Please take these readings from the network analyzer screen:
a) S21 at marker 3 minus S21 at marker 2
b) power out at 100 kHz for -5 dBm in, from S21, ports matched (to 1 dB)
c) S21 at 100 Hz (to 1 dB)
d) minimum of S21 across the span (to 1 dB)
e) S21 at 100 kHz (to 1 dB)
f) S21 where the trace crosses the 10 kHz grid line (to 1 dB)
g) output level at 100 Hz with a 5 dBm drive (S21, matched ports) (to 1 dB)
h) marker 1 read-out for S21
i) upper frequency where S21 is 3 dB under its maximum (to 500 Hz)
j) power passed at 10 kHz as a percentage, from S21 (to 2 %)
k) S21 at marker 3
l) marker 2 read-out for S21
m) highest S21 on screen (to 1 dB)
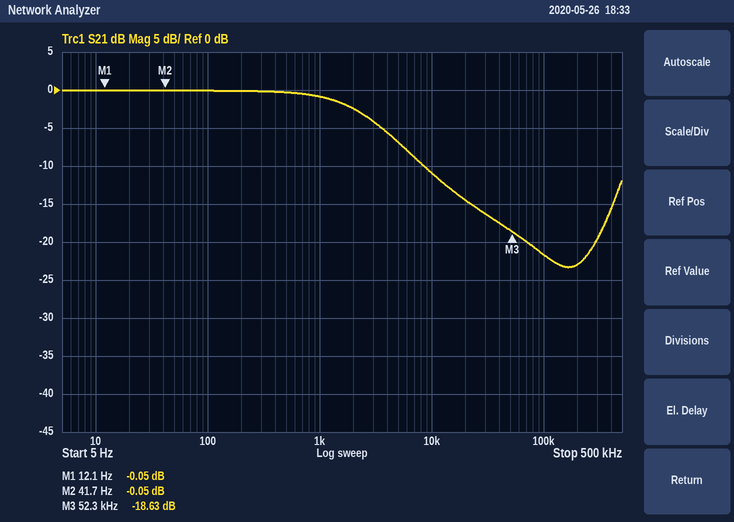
-18.58 dB
-27 dBm
0 dB
-23 dB
-22 dB
-11 dB
5 dBm
-0.05 dB
2.5 kHz
8 %
-18.63 dB
-0.05 dB
0 dB
